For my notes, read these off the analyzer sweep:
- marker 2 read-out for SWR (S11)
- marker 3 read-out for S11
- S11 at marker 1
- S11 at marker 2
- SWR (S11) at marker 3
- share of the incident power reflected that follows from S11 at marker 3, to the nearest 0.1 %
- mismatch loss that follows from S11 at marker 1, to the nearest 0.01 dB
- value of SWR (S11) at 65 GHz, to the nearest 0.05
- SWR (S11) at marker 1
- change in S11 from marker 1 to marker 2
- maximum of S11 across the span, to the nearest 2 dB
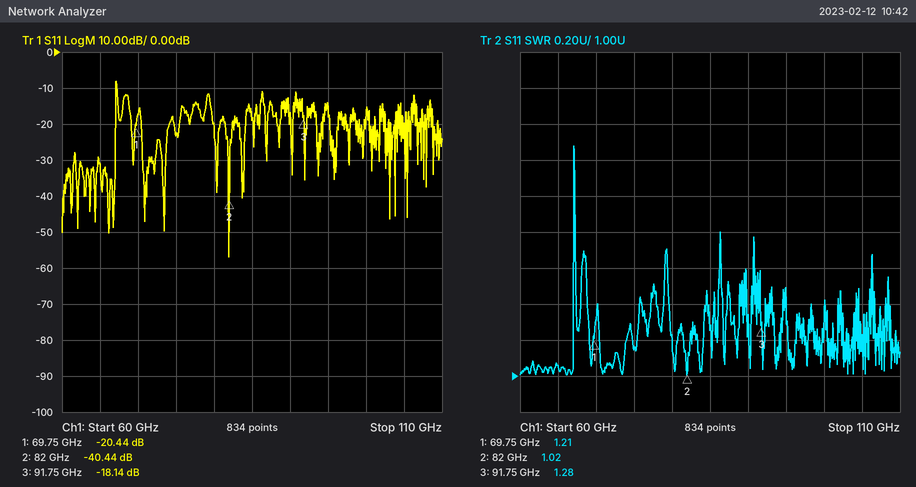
1.02
-18.14 dB
-20.44 dB
-40.44 dB
1.28
1.5 %
0.04 dB
1.05
1.21
-20.00 dB
-8 dB
